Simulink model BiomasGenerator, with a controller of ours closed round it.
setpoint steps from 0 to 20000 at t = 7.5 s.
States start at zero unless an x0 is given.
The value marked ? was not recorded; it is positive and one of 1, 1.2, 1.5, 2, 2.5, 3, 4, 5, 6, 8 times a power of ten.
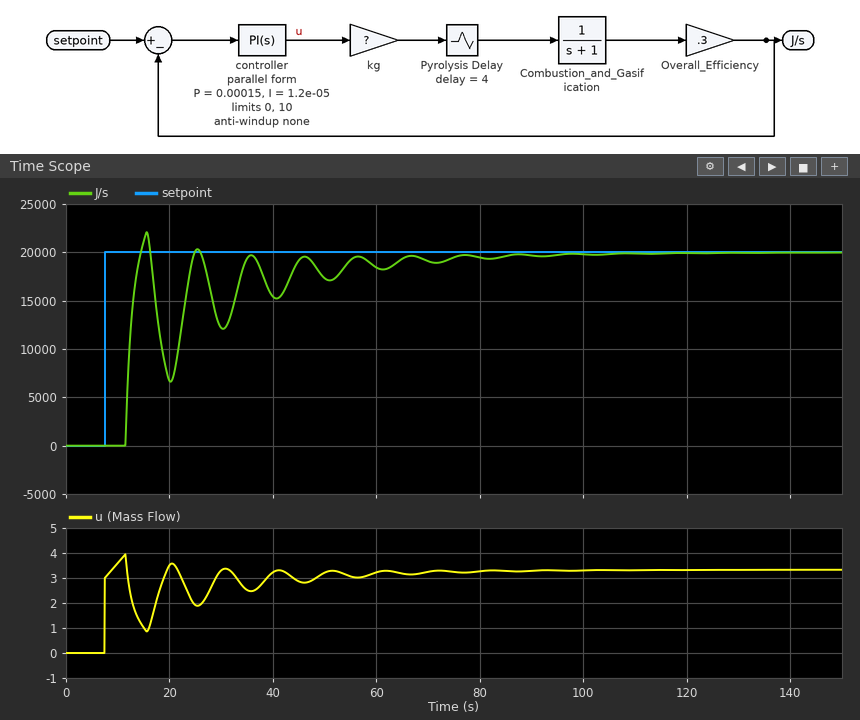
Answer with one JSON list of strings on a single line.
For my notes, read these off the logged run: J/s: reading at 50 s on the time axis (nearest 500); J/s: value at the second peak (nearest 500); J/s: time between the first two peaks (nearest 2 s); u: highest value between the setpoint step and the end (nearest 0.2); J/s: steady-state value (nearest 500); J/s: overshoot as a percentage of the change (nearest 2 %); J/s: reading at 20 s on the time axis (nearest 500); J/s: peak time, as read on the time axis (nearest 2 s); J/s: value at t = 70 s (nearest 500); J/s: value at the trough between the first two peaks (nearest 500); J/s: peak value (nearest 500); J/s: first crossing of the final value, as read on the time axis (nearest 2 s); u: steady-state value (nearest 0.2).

["17500", "20500", "10 s", "4.0", "20000", "10 %", "6500", "16 s", "19000", "6500", "22000", "14 s", "3.4"]
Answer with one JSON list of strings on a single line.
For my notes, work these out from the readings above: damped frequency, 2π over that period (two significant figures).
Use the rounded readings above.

["0.63 rad/s"]
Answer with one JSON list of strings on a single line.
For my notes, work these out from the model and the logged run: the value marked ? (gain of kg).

["20000"]
